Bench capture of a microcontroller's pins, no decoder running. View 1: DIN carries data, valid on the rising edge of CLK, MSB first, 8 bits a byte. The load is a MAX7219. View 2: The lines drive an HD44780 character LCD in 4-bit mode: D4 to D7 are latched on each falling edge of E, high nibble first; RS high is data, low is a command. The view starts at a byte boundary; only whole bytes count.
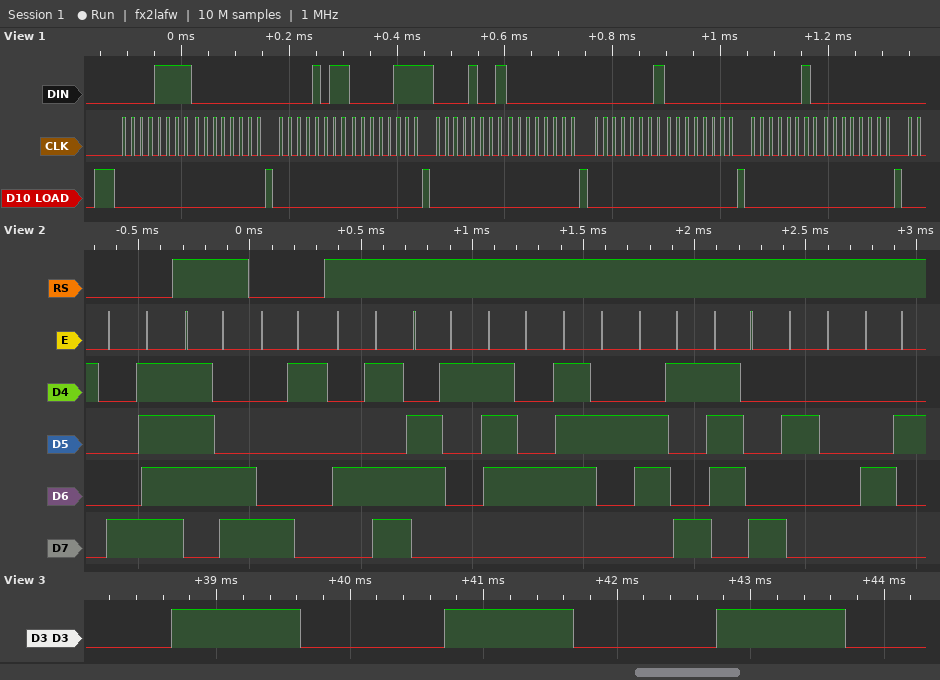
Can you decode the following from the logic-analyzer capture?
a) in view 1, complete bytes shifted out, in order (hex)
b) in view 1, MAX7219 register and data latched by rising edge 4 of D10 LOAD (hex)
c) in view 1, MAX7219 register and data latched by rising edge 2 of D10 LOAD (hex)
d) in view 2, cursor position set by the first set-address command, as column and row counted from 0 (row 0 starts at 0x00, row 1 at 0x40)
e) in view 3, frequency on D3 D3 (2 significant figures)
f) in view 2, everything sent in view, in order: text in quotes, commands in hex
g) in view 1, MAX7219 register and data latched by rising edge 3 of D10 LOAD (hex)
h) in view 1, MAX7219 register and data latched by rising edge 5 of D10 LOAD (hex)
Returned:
0F 00 0B 07 09 00 01 00 02 00
register 0x9, data 0x00
register 0xF, data 0x00
column 15, row 0
490 Hz
0x8F "|" 0x81 "Matrix B"
register 0xB, data 0x07
register 0x1, data 0x00
